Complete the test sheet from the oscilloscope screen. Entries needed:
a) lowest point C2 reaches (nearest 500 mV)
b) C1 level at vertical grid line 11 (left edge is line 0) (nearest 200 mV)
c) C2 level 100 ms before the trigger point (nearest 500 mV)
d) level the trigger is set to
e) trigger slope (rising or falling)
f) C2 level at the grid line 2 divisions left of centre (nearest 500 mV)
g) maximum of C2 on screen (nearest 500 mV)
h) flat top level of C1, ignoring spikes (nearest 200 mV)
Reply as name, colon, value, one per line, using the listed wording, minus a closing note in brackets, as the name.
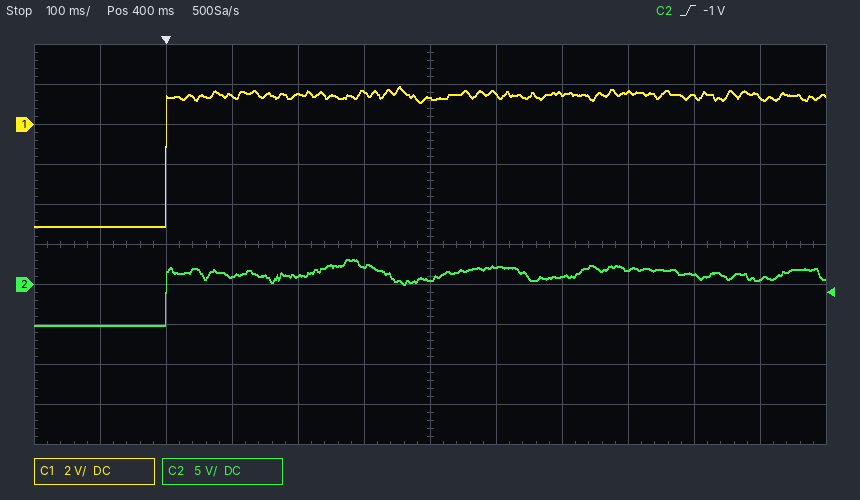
lowest point C2 reaches: -5.0 V
C1 level at vertical grid line 11 (left edge is line 0): 1.4 V
C2 level 100 ms before the trigger point: -5.0 V
level the trigger is set to: -1 V
trigger slope: rising
C2 level at the grid line 2 divisions left of centre: 1.0 V
maximum of C2 on screen: 3.0 V
flat top level of C1, ignoring spikes: 1.4 V
